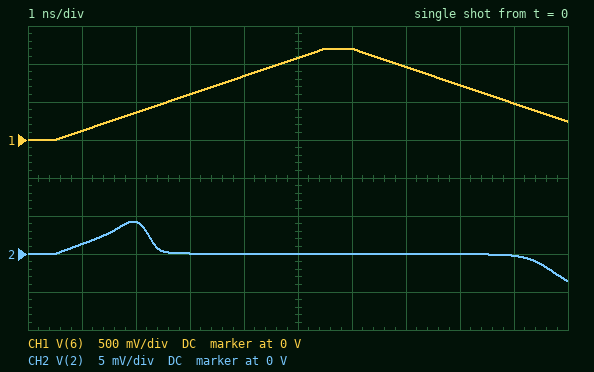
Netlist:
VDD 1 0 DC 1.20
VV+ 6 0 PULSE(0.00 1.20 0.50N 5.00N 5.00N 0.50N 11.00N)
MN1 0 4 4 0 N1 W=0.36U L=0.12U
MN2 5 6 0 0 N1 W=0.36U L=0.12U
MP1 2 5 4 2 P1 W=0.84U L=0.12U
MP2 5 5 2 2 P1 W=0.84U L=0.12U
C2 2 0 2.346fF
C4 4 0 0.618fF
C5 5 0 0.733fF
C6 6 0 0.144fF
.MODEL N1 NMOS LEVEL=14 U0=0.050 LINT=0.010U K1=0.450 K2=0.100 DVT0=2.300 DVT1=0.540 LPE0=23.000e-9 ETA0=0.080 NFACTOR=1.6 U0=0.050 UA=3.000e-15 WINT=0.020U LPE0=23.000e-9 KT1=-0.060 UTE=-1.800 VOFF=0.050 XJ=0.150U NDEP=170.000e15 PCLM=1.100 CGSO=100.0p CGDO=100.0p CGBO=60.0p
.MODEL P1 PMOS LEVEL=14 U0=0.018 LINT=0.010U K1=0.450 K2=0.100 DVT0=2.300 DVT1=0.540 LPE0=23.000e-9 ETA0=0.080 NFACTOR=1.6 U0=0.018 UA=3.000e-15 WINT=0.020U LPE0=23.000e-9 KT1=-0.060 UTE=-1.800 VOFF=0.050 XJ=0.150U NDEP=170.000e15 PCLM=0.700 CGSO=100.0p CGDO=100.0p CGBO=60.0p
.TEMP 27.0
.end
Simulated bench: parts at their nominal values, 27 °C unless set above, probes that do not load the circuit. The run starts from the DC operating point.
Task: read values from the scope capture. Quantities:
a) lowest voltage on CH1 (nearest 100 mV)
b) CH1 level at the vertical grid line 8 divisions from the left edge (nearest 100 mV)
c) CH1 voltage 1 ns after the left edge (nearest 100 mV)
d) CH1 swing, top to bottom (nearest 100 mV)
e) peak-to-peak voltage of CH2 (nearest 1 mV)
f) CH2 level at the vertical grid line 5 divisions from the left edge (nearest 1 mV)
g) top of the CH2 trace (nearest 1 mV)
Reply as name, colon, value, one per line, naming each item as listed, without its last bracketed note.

lowest voltage on CH1: 0 V
CH1 level at the vertical grid line 8 divisions from the left edge: 700 mV
CH1 voltage 1 ns after the left edge: 100 mV
CH1 swing, top to bottom: 1.2 V
peak-to-peak voltage of CH2: 8 mV
CH2 level at the vertical grid line 5 divisions from the left edge: 0 V
top of the CH2 trace: 4 mV
